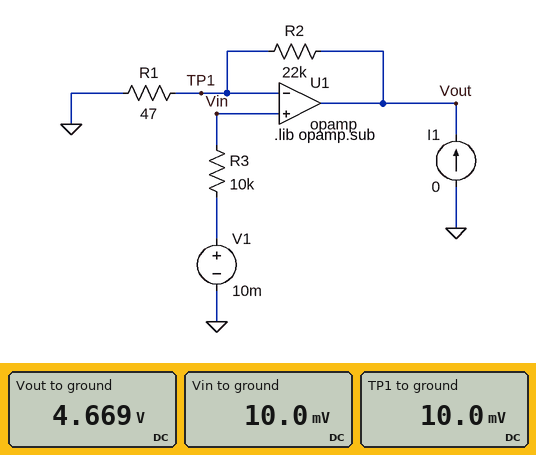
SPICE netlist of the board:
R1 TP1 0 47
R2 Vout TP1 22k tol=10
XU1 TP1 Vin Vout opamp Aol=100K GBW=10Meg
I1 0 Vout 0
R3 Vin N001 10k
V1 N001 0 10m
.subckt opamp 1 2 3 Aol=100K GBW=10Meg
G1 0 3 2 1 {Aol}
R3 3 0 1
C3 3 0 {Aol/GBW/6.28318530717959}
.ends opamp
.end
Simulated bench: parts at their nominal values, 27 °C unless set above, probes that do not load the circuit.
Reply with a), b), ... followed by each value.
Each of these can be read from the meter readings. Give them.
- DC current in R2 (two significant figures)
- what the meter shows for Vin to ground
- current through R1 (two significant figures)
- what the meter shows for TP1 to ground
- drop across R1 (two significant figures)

a) 210 µA
b) 10.0 mV
c) 210 µA
d) 10.0 mV
e) 10 mV
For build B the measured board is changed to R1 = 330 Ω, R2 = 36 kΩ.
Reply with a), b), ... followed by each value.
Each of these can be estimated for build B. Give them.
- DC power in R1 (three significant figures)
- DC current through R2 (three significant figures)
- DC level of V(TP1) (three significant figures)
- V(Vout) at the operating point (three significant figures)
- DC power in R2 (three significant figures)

a) 302 nW
b) 30.3 µA
c) 9.99 mV
d) 1.10 V
e) 33.0 µW
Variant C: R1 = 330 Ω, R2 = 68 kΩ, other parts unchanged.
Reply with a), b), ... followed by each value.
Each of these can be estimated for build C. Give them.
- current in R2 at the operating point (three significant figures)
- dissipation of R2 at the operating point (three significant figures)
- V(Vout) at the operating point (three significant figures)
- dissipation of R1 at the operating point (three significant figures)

a) 30.2 µA
b) 62.2 µW
c) 2.07 V
d) 302 nW
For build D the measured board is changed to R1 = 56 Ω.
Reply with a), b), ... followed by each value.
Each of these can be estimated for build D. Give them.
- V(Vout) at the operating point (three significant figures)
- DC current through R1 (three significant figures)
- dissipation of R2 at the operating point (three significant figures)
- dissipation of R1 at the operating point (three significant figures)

a) 3.92 V
b) 178 µA
c) 696 µW
d) 1.77 µW
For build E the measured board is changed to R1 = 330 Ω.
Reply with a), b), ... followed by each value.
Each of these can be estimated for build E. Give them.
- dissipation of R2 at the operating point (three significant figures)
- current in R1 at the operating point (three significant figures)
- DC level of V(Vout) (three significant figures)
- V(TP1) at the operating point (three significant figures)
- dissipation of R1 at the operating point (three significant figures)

a) 20.2 µW
b) 30.3 µA
c) 676 mV
d) 9.99 mV
e) 303 nW
